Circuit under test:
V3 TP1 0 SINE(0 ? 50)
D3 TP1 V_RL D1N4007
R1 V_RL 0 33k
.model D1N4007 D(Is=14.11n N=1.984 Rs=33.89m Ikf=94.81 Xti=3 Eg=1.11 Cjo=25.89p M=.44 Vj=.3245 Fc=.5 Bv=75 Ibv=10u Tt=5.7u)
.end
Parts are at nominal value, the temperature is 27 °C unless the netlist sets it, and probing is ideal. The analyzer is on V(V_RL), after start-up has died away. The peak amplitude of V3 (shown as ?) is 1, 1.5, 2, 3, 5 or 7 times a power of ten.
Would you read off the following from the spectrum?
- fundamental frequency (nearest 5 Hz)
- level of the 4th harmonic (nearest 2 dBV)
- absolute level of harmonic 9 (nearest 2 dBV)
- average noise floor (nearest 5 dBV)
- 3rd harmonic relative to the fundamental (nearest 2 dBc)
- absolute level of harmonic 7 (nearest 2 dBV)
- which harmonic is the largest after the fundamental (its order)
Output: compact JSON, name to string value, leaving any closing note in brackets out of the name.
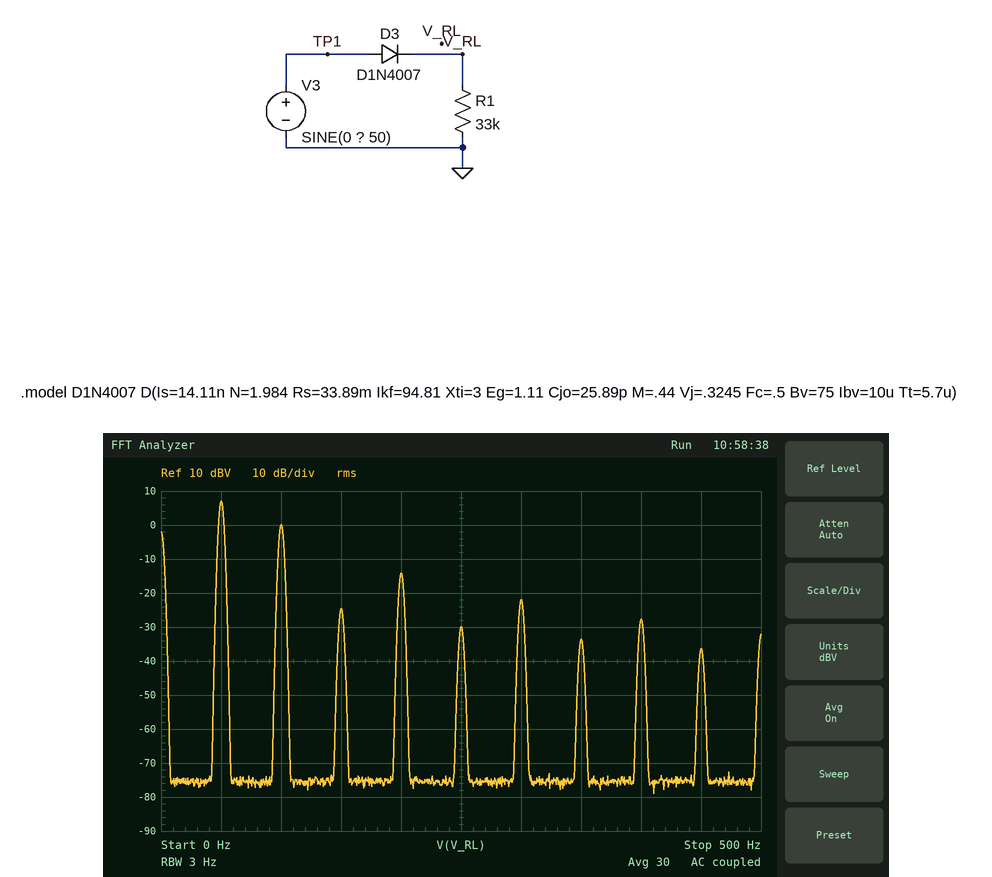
{"fundamental frequency": "50 Hz", "level of the 4th harmonic": "-14 dBV", "absolute level of harmonic 9": "-36 dBV", "average noise floor": "-75 dBV", "3rd harmonic relative to the fundamental": "-32 dBc", "absolute level of harmonic 7": "-34 dBV", "which harmonic is the largest after the fundamental": "2"}
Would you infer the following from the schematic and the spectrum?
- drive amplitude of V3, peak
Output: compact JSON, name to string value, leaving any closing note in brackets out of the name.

{"drive amplitude of V3, peak": "7 V"}
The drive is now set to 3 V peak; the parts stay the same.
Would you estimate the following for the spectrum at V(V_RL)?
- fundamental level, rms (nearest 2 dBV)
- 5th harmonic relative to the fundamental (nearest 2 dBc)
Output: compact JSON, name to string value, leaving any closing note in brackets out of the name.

{"fundamental level, rms": "-2 dBV", "5th harmonic relative to the fundamental": "-30 dBc"}
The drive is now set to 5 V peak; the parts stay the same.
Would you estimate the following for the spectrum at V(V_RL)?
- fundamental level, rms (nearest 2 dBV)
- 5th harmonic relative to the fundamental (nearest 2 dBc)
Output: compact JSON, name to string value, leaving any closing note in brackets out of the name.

{"fundamental level, rms": "4 dBV", "5th harmonic relative to the fundamental": "-34 dBc"}
